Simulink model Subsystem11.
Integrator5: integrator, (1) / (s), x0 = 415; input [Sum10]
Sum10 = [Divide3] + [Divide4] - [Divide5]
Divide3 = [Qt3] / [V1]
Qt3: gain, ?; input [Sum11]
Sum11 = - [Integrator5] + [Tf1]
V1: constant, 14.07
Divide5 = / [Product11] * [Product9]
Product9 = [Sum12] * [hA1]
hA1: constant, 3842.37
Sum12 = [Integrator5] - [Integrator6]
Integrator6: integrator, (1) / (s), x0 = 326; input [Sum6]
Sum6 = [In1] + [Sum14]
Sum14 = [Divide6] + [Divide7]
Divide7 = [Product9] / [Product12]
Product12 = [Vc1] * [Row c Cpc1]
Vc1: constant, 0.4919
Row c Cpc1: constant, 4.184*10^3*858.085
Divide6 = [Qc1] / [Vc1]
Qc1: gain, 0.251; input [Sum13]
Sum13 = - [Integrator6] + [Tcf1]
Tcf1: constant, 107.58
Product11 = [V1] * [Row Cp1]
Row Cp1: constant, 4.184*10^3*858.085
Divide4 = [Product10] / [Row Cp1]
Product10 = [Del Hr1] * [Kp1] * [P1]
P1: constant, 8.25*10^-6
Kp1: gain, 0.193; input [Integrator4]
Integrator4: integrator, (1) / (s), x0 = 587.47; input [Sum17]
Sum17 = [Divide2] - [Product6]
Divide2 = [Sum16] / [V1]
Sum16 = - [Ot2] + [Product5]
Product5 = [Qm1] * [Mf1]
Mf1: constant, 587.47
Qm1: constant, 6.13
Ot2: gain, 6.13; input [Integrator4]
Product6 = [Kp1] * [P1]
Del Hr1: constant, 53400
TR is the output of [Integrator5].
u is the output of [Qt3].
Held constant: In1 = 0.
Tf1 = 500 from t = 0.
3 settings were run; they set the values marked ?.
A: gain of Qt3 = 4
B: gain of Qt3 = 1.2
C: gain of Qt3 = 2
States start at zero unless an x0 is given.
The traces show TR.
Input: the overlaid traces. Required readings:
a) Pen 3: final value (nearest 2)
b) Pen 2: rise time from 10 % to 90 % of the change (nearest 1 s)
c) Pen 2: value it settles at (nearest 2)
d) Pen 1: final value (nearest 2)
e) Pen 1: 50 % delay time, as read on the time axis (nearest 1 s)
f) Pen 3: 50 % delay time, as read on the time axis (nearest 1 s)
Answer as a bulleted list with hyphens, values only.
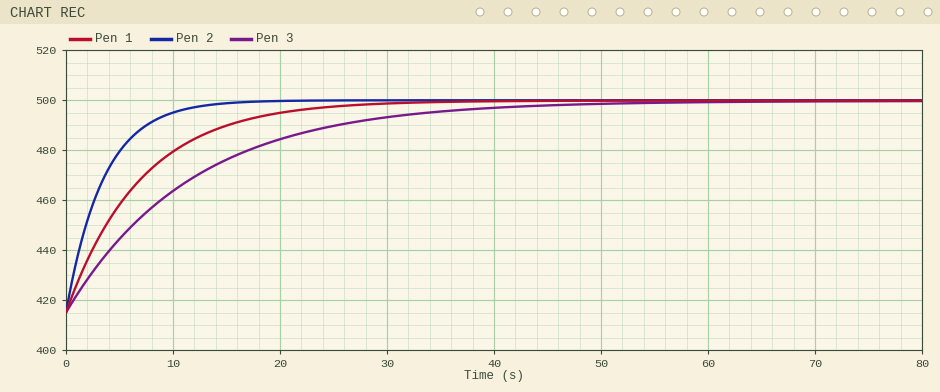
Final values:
- 500
- 8 s
- 500
- 500
- 5 s
- 8 s
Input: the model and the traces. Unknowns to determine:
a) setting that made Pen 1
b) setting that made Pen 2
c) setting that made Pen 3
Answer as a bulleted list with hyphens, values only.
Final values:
- C
- A
- B
